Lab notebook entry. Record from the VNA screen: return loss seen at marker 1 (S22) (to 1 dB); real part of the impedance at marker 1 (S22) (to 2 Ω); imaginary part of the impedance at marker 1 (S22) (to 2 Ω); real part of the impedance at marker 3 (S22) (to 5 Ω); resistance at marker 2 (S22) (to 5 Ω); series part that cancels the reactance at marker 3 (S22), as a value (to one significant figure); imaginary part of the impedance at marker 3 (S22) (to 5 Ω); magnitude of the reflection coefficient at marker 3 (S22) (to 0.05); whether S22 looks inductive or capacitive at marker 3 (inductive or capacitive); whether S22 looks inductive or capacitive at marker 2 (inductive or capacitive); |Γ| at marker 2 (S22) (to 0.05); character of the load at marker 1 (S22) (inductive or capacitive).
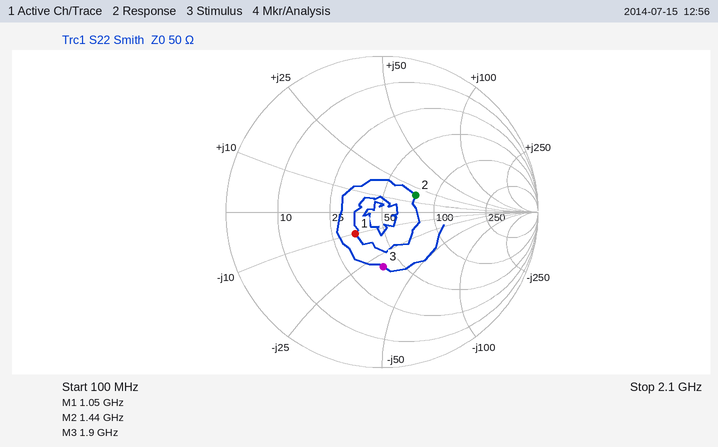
13 dB
34 Ω
-10 Ω
40 Ω
75 Ω
3 nH
-30 Ω
0.35
capacitive
inductive
0.25
capacitive
